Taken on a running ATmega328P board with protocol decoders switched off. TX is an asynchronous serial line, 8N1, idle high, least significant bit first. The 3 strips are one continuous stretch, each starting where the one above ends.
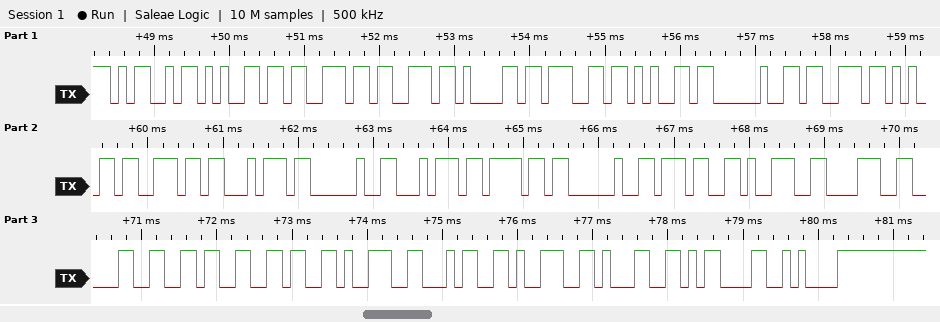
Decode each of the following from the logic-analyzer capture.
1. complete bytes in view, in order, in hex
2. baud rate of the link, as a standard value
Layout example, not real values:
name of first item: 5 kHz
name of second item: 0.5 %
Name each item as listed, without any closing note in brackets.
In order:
complete bytes in view, in order, in hex: 4D 65 73 73 61 67 65 20 73 65 6E 74 20 74 6F 20 37 39 38 30 36 36 39 34 39 31 0D 0A
baud rate of the link, as a standard value: 9600 baud
